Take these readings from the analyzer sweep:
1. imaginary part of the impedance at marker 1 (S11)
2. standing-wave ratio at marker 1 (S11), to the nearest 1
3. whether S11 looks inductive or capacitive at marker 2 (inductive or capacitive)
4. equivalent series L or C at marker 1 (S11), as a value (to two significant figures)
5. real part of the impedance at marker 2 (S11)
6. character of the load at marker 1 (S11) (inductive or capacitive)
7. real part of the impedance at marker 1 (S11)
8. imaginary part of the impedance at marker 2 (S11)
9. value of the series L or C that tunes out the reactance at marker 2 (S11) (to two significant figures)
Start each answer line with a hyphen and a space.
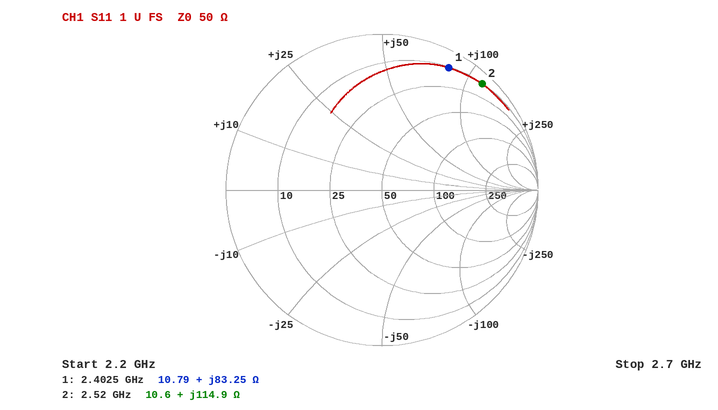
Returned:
- +83.25 Ω
- 18
- inductive
- 5.5 nH
- 10.6 Ω
- inductive
- 10.79 Ω
- +114.9 Ω
- 550 fF
